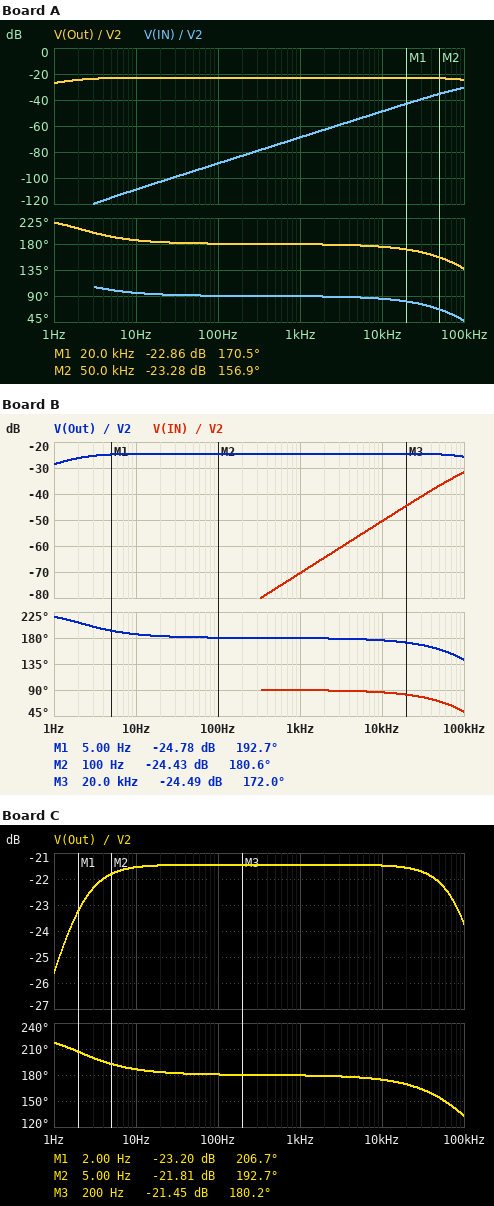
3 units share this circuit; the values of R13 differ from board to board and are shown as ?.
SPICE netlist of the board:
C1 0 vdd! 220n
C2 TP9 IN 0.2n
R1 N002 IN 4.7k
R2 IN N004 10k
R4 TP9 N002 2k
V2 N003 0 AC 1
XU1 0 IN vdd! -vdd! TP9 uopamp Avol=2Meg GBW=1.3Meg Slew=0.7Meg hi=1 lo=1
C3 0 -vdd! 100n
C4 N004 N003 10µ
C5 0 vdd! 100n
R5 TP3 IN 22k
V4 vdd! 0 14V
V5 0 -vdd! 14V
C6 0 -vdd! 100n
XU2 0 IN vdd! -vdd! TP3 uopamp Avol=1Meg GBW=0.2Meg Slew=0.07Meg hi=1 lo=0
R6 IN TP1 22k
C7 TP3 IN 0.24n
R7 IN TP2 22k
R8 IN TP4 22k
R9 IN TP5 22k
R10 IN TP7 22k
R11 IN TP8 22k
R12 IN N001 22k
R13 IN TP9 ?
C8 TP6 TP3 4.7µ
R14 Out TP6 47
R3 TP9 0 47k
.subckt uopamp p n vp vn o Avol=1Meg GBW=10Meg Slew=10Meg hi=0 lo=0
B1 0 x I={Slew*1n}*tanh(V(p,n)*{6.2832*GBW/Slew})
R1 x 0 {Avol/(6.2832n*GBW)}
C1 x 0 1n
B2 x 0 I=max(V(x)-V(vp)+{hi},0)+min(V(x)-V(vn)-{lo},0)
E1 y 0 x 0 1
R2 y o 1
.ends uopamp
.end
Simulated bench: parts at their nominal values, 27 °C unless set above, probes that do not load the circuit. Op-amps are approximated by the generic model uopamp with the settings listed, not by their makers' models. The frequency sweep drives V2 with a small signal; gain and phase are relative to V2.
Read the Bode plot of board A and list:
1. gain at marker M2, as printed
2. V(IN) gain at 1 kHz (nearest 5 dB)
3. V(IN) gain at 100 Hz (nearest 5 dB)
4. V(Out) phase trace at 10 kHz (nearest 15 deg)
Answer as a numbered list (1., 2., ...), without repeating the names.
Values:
1. -23.28 dB
2. -70 dB
3. -90 dB
4. 180 deg
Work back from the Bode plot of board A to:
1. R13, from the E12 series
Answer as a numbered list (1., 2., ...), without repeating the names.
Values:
1. 18 kΩ
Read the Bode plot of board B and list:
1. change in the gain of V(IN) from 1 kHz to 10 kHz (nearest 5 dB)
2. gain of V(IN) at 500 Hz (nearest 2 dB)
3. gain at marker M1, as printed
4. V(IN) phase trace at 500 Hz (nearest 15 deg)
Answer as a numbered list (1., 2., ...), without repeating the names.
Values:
1. 20 dB
2. -76 dB
3. -24.78 dB
4. 90 deg
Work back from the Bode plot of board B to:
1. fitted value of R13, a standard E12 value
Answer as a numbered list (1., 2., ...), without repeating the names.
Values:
1. 10 kΩ
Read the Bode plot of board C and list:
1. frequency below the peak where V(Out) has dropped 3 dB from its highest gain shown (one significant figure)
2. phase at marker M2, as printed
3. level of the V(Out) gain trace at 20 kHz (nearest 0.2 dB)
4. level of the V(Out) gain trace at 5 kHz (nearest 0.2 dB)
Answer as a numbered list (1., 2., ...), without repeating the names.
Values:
1. 1 Hz
2. 192.7 deg
3. -21.6 dB
4. -21.4 dB
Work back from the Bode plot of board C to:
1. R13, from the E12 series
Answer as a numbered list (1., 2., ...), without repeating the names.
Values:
1. 39 kΩ
